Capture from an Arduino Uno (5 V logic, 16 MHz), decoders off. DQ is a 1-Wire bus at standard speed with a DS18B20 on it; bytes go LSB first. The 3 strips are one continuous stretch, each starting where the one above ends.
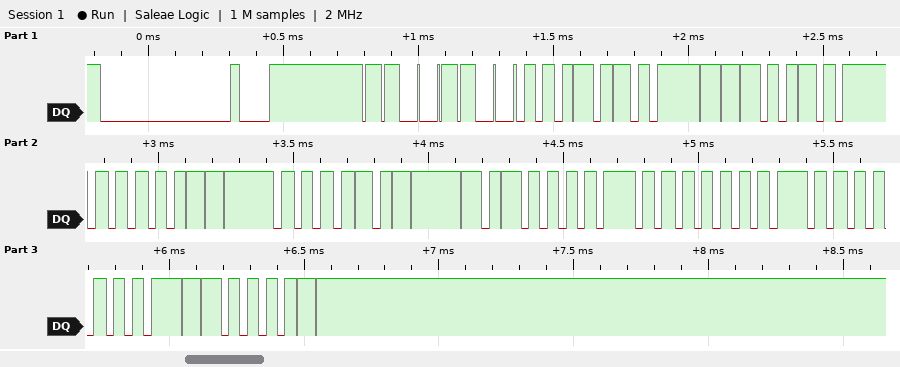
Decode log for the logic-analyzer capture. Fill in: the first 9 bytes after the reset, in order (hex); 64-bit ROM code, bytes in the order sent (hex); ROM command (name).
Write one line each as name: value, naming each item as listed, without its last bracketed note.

the first 9 bytes after the reset, in order: 33 28 27 E0 D0 05 00 00 C3
64-bit ROM code, bytes in the order sent: 28 27 E0 D0 05 00 00 C3
ROM command: Read ROM
